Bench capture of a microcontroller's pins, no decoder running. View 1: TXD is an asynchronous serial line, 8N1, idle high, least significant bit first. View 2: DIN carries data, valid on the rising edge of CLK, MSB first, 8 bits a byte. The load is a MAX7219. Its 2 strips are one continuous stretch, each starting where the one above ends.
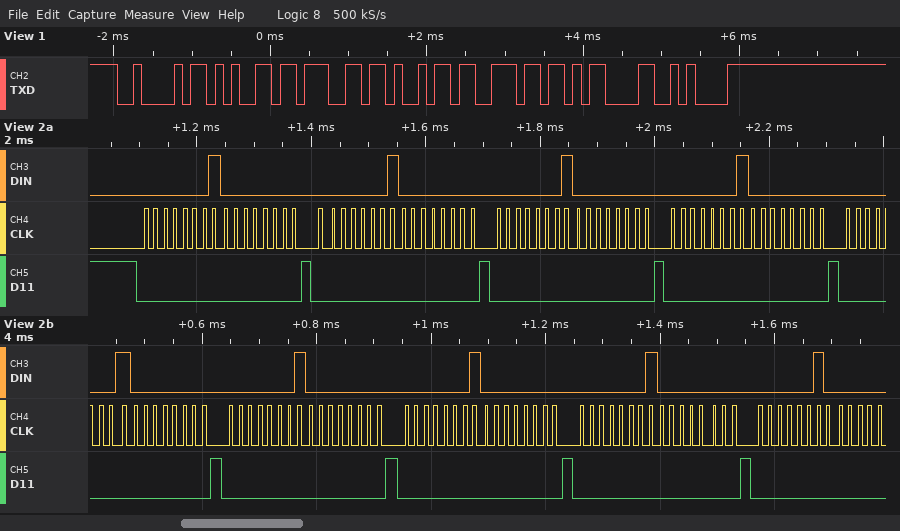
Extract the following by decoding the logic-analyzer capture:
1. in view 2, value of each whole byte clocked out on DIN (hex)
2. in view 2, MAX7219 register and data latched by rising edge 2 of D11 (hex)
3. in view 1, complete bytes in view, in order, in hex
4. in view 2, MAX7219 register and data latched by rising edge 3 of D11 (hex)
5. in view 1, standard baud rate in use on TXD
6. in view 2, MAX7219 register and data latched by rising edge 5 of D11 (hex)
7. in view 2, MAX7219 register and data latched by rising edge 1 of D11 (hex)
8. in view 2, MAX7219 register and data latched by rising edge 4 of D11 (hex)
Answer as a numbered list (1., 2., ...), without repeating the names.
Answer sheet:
1. 01 00 01 00 01 00 01 00 01 00 01 00 01 00 01 00 02
2. register 0x1, data 0x00
3. 42 65 67 69 6E 0D 0A
4. register 0x1, data 0x00
5. 9600 baud
6. register 0x1, data 0x00
7. register 0x1, data 0x00
8. register 0x1, data 0x00
